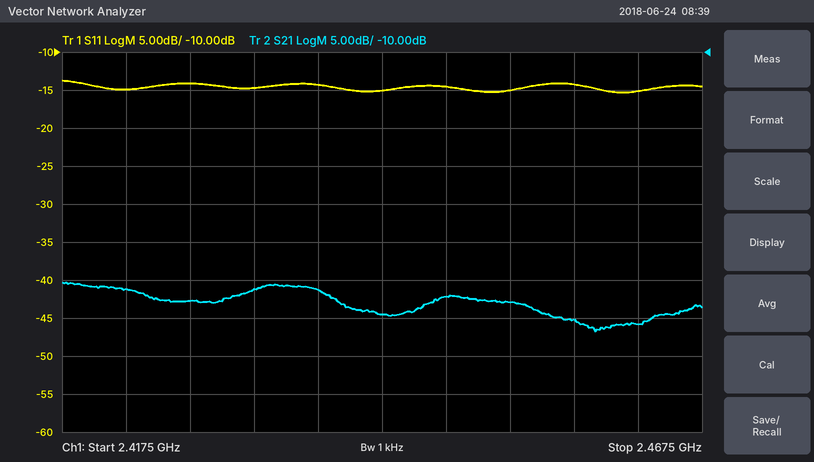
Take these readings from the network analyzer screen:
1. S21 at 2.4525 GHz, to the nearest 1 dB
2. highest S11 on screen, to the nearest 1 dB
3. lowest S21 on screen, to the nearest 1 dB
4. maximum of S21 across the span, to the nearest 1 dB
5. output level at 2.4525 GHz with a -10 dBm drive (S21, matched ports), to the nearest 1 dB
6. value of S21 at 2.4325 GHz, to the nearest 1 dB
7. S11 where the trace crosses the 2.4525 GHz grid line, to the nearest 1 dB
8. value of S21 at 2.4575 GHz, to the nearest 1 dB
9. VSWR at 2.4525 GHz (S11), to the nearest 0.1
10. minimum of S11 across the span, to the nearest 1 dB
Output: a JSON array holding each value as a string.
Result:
["-43 dB", "-14 dB", "-47 dB", "-40 dB", "-53 dBm", "-41 dB", "-15 dB", "-45 dB", "1.4", "-15 dB"]
